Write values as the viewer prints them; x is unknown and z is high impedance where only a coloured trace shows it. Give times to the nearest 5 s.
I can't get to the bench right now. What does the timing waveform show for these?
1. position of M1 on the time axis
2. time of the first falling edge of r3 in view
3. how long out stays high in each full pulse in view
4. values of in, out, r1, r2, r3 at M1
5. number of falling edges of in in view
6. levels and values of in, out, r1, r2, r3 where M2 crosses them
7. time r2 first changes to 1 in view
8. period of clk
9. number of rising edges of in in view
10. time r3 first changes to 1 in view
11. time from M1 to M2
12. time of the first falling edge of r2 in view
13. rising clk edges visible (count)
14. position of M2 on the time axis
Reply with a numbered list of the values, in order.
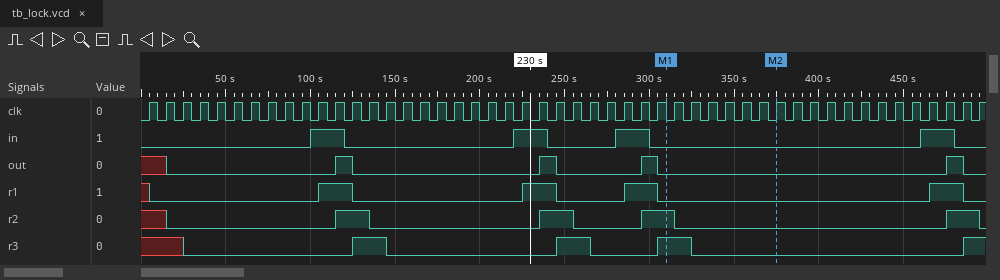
1. 310 s
2. 145 s
3. 10 s, 10 s, 10 s, 10 s
4. in=0, out=0, r1=0, r2=1, r3=1
5. 4
6. in=0, out=0, r1=0, r2=0, r3=0
7. 115 s
8. 10 s
9. 4
10. 125 s
11. 65 s
12. 135 s
13. 50
14. 375 s
